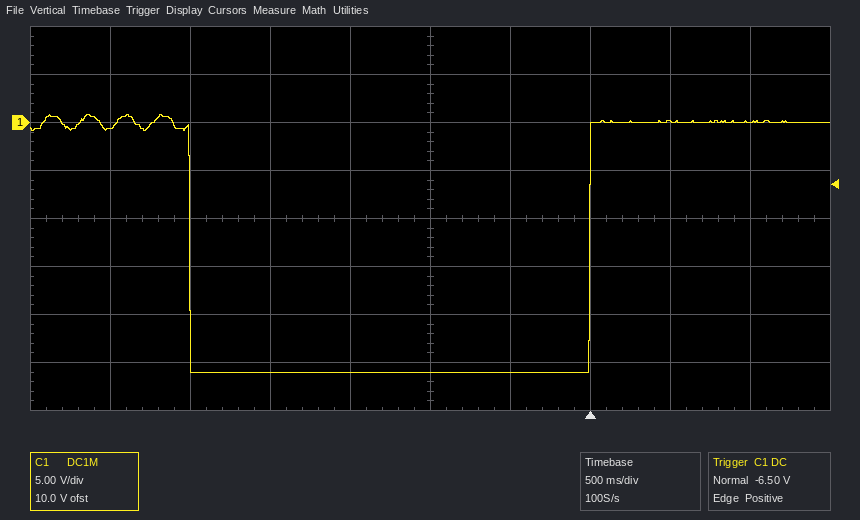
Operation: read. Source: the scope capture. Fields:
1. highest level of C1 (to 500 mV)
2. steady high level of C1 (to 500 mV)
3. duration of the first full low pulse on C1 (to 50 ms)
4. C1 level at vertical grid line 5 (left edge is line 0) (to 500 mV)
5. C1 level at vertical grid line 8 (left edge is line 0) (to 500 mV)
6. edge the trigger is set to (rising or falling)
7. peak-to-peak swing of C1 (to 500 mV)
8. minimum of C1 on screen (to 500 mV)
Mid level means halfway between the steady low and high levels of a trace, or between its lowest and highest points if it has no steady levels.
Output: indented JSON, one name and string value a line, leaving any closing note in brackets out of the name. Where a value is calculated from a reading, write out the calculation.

{
  "highest level of C1": "1.0 V",
  "steady high level of C1": "0.0 V",
  "duration of the first full low pulse on C1": "2.50 s",
  "C1 level at vertical grid line 5 (left edge is line 0)": "-26.0 V",
  "C1 level at vertical grid line 8 (left edge is line 0)": "0.0 V",
  "edge the trigger is set to": "rising",
  "peak-to-peak swing of C1": "1.0 V − (-26.0 V) = 27.0 V",
  "minimum of C1 on screen": "-26.0 V"
}
